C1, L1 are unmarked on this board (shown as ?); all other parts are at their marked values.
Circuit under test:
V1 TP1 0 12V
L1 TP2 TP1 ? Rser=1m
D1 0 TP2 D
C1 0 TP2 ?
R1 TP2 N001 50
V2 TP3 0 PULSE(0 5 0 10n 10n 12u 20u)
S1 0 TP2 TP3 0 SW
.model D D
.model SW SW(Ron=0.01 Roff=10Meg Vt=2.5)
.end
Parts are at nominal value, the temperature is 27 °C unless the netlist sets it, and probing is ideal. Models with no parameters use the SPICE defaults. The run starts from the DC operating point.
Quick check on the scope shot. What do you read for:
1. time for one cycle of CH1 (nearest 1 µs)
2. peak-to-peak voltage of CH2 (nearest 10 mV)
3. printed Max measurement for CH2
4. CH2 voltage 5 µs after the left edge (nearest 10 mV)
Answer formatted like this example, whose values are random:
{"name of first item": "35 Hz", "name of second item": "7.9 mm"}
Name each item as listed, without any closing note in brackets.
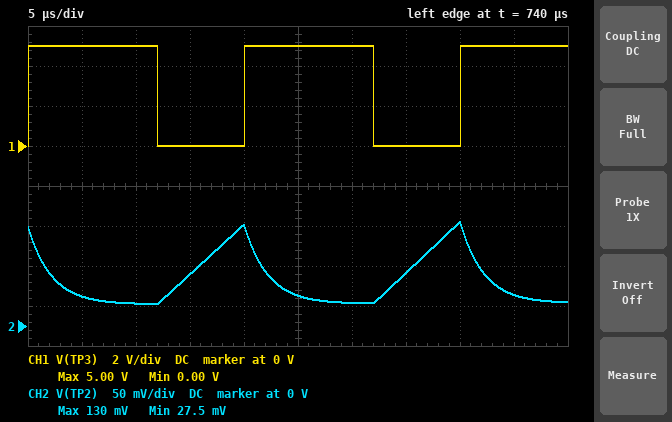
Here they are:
{"time for one cycle of CH1": "20 µs", "peak-to-peak voltage of CH2": "100 mV", "printed Max measurement for CH2": "130 mV", "CH2 voltage 5 µs after the left edge": "40 mV"}
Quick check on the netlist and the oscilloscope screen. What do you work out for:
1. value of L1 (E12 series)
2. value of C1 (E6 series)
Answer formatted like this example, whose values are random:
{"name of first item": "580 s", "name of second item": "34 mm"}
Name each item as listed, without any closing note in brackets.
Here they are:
{"value of L1": "3.3 mH", "value of C1": "220 µF"}
